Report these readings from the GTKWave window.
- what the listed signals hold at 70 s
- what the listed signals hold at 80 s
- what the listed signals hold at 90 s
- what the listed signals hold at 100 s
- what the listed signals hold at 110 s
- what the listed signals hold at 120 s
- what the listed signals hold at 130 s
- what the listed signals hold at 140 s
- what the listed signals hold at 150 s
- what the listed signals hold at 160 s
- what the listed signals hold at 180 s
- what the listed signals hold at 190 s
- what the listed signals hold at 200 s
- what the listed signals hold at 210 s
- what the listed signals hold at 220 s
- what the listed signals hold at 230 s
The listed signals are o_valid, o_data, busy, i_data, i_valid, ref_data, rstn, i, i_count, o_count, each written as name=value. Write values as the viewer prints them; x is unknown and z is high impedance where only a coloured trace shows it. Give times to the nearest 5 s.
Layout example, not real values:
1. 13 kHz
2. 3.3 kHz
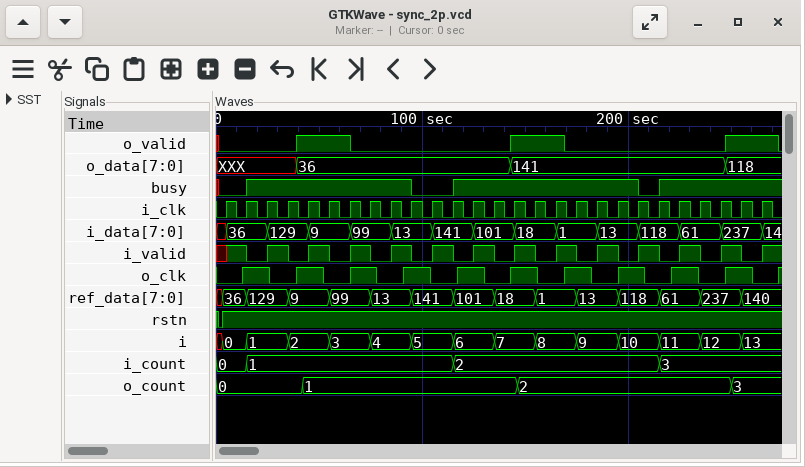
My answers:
1. o_valid=0, o_data=36, busy=1, i_data=99, i_valid=1, ref_data=99, rstn=1, i=3, i_count=1, o_count=1
2. o_valid=0, o_data=36, busy=1, i_data=99, i_valid=0, ref_data=13, rstn=1, i=4, i_count=1, o_count=1
3. o_valid=0, o_data=36, busy=1, i_data=13, i_valid=1, ref_data=13, rstn=1, i=4, i_count=1, o_count=1
4. o_valid=0, o_data=36, busy=0, i_data=13, i_valid=0, ref_data=141, rstn=1, i=5, i_count=1, o_count=1
5. o_valid=0, o_data=36, busy=0, i_data=141, i_valid=1, ref_data=141, rstn=1, i=5, i_count=1, o_count=1
6. o_valid=0, o_data=36, busy=1, i_data=141, i_valid=0, ref_data=101, rstn=1, i=6, i_count=2, o_count=1
7. o_valid=0, o_data=36, busy=1, i_data=101, i_valid=1, ref_data=101, rstn=1, i=6, i_count=2, o_count=1
8. o_valid=0, o_data=36, busy=1, i_data=101, i_valid=0, ref_data=18, rstn=1, i=7, i_count=2, o_count=1
9. o_valid=1, o_data=141, busy=1, i_data=18, i_valid=1, ref_data=18, rstn=1, i=7, i_count=2, o_count=2
10. o_valid=1, o_data=141, busy=1, i_data=18, i_valid=0, ref_data=1, rstn=1, i=8, i_count=2, o_count=2
11. o_valid=0, o_data=141, busy=1, i_data=1, i_valid=0, ref_data=13, rstn=1, i=9, i_count=2, o_count=2
12. o_valid=0, o_data=141, busy=1, i_data=13, i_valid=1, ref_data=13, rstn=1, i=9, i_count=2, o_count=2
13. o_valid=0, o_data=141, busy=1, i_data=13, i_valid=0, ref_data=118, rstn=1, i=10, i_count=2, o_count=2
14. o_valid=0, o_data=141, busy=0, i_data=118, i_valid=1, ref_data=118, rstn=1, i=10, i_count=2, o_count=2
15. o_valid=0, o_data=141, busy=1, i_data=118, i_valid=0, ref_data=61, rstn=1, i=11, i_count=3, o_count=2
16. o_valid=0, o_data=141, busy=1, i_data=61, i_valid=1, ref_data=61, rstn=1, i=11, i_count=3, o_count=2
